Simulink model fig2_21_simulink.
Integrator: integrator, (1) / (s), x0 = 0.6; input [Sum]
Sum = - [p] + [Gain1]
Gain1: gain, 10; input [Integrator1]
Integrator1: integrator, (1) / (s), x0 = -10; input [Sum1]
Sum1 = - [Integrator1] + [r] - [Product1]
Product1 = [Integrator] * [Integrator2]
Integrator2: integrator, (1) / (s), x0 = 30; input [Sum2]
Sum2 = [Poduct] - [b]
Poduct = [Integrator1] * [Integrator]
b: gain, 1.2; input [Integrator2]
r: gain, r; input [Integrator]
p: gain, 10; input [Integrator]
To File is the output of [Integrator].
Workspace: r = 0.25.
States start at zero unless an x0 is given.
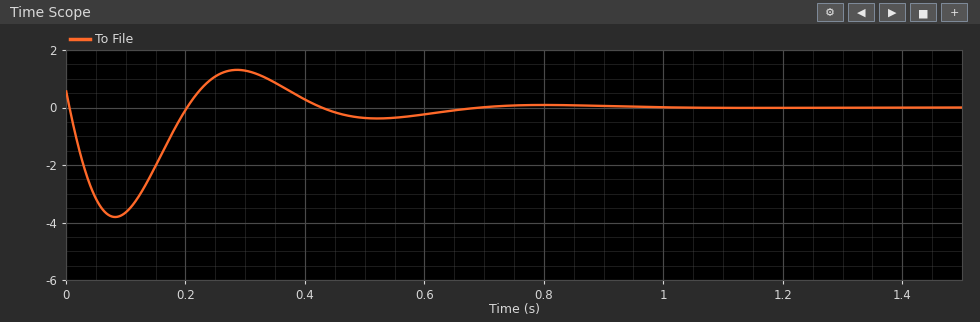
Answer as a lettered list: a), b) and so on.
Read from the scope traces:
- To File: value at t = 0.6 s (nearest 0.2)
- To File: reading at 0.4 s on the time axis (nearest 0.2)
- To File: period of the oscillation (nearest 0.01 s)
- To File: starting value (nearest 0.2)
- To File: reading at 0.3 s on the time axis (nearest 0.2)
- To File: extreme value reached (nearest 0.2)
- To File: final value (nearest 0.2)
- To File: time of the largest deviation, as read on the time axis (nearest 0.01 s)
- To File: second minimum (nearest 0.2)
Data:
a) -0.2
b) 0.2
c) 0.44 s
d) 0.6
e) 1.2
f) -3.8
g) 0.0
h) 0.08 s
i) -0.4
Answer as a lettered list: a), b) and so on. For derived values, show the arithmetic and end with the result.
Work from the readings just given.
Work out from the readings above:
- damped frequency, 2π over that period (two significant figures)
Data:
a) 2π / 0.44 = 14 rad/s
